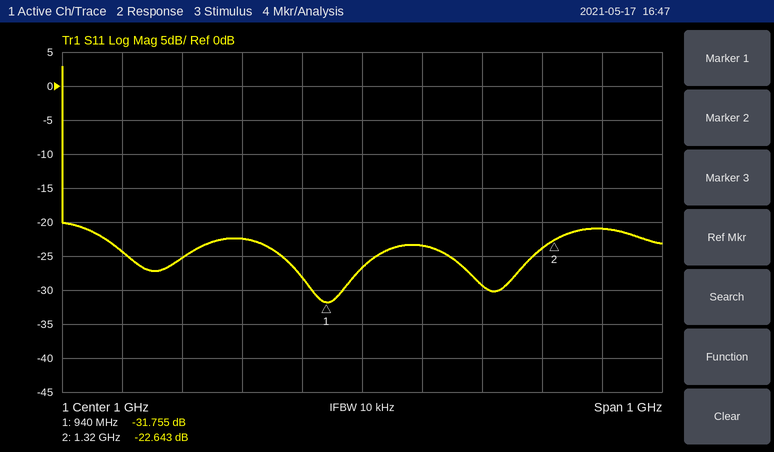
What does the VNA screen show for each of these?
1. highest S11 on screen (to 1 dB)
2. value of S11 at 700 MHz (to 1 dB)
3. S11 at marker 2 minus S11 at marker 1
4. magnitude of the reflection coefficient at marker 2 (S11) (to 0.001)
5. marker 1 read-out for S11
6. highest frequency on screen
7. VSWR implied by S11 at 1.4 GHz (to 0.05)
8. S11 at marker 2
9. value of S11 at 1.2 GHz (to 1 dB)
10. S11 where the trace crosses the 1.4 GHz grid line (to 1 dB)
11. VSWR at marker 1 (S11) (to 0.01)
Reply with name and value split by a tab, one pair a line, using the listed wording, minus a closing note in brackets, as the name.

highest S11 on screen	3 dB
value of S11 at 700 MHz	-25 dB
S11 at marker 2 minus S11 at marker 1	9.112 dB
magnitude of the reflection coefficient at marker 2 (S11)	0.074
marker 1 read-out for S11	-31.755 dB
highest frequency on screen	1.5 GHz
VSWR implied by S11 at 1.4 GHz	1.20
S11 at marker 2	-22.643 dB
value of S11 at 1.2 GHz	-29 dB
S11 where the trace crosses the 1.4 GHz grid line	-21 dB
VSWR at marker 1 (S11)	1.05
